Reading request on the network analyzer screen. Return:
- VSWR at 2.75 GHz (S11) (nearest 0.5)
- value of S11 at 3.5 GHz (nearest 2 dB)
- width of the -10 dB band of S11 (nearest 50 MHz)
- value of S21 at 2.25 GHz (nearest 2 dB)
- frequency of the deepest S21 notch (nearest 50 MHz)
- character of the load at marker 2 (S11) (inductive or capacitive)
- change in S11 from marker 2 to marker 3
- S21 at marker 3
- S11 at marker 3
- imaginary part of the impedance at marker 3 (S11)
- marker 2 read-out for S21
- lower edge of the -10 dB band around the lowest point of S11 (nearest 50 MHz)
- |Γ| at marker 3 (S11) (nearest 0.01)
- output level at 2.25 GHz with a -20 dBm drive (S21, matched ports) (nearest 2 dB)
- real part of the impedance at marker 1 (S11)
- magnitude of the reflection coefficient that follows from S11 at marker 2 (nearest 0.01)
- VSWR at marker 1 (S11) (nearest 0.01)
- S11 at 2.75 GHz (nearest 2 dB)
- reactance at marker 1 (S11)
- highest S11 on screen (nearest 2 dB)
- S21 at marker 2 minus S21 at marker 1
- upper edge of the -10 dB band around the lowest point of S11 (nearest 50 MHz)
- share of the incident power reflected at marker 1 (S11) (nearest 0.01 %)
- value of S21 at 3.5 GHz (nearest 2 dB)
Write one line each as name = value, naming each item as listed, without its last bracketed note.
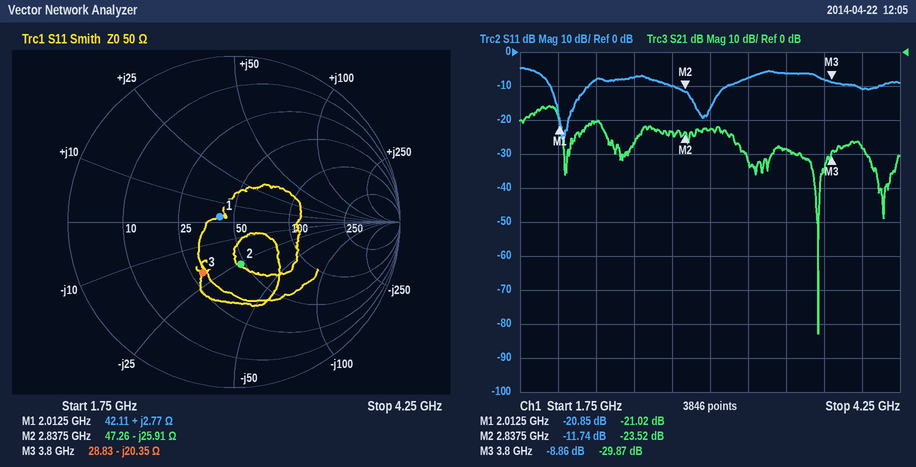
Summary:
VSWR at 2.75 GHz (S11) = 2.0
value of S11 at 3.5 GHz = -6 dB
width of the -10 dB band of S11 = 250 MHz
value of S21 at 2.25 GHz = -20 dB
frequency of the deepest S21 notch = 3.70 GHz
character of the load at marker 2 (S11) = capacitive
change in S11 from marker 2 to marker 3 = 2.88 dB
S21 at marker 3 = -29.87 dB
S11 at marker 3 = -8.86 dB
imaginary part of the impedance at marker 3 = -20.35 Ω
marker 2 read-out for S21 = -23.52 dB
lower edge of the -10 dB band around the lowest point of S11 = 1.95 GHz
|Γ| at marker 3 (S11) = 0.36
output level at 2.25 GHz with a -20 dBm drive (S21, matched ports) = -40 dBm
real part of the impedance at marker 1 = 42.11 Ω
magnitude of the reflection coefficient that follows from S11 at marker 2 = 0.26
VSWR at marker 1 (S11) = 1.20
S11 at 2.75 GHz = -10 dB
reactance at marker 1 = +2.77 Ω
highest S11 on screen = -4 dB
S21 at marker 2 minus S21 at marker 1 = -2.50 dB
upper edge of the -10 dB band around the lowest point of S11 = 2.20 GHz
share of the incident power reflected at marker 1 (S11) = 0.82 %
value of S21 at 3.5 GHz = -28 dB
